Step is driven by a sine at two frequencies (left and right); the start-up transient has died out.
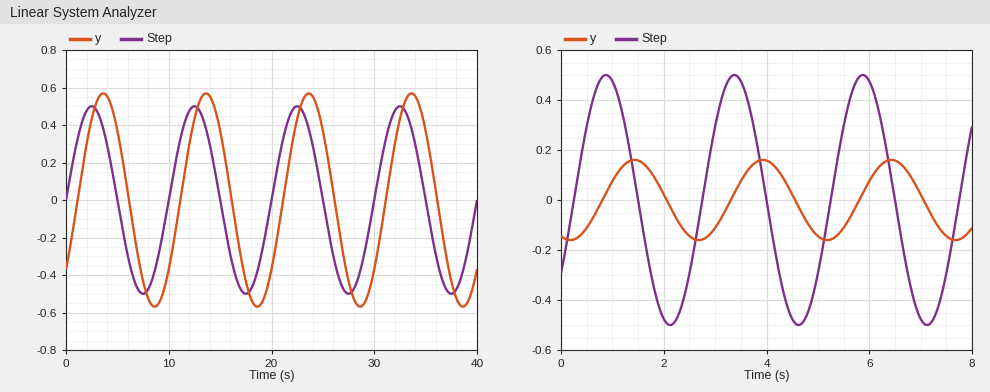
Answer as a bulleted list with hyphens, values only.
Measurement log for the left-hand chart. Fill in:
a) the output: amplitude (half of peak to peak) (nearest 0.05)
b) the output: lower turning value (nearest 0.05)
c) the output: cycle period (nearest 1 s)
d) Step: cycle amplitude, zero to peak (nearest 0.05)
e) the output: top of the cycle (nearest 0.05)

- 0.55
- -0.55
- 10 s
- 0.50
- 0.55
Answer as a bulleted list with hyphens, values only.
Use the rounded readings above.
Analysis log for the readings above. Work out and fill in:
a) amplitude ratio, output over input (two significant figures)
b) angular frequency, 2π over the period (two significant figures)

- 1.1
- 0.63 rad/s
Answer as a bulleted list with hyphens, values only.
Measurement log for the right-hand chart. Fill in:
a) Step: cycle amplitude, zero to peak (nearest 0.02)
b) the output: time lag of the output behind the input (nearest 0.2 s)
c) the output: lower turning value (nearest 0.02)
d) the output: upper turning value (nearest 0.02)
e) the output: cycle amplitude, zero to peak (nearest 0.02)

- 0.50
- 0.6 s
- -0.16
- 0.16
- 0.16
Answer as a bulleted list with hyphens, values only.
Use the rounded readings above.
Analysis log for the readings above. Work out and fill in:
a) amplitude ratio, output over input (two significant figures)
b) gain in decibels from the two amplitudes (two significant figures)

- 0.32
- -9.9 dB
